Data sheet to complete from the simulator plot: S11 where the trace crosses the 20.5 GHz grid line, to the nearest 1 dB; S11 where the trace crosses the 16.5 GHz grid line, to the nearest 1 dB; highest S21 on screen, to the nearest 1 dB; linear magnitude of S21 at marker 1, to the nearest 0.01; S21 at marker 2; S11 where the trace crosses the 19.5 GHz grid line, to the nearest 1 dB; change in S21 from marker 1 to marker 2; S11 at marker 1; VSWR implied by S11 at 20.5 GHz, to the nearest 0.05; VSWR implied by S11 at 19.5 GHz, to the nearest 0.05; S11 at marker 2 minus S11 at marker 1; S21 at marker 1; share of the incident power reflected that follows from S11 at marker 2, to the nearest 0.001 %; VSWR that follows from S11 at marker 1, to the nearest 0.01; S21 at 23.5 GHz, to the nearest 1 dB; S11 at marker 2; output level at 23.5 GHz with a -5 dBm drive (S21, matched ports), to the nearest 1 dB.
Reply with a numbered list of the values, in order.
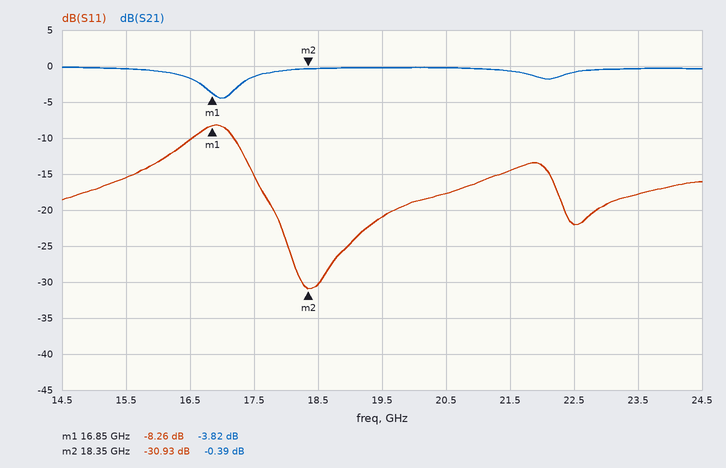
1. -18 dB
2. -10 dB
3. 0 dB
4. 0.64
5. -0.39 dB
6. -21 dB
7. 3.43 dB
8. -8.26 dB
9. 1.30
10. 1.20
11. -22.67 dB
12. -3.82 dB
13. 0.081 %
14. 2.26
15. 0 dB
16. -30.93 dB
17. -5 dBm
